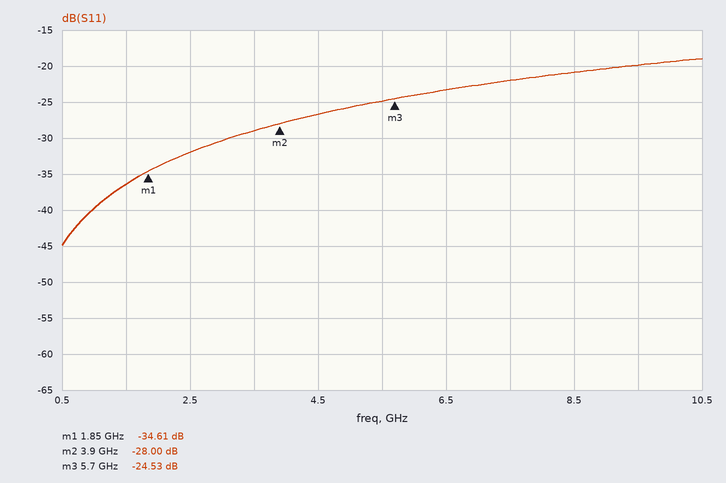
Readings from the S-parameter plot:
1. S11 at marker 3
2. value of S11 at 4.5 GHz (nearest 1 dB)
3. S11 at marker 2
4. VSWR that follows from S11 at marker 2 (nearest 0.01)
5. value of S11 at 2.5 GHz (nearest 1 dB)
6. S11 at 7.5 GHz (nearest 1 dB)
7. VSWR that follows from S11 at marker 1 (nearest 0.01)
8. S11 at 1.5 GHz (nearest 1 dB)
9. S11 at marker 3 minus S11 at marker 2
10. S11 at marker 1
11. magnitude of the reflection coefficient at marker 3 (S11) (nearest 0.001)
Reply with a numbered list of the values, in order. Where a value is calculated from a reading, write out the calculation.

1. -24.53 dB
2. -27 dB
3. -28.00 dB
4. (1 + 0.0398)/(1 − 0.0398) ≈ 1.08
5. -32 dB
6. -22 dB
7. (1 + 0.0186)/(1 − 0.0186) ≈ 1.04
8. -36 dB
9. -24.53 − (-28) = 3.47 dB
10. -34.61 dB
11. 10^(-24.53/20) ≈ 0.059
